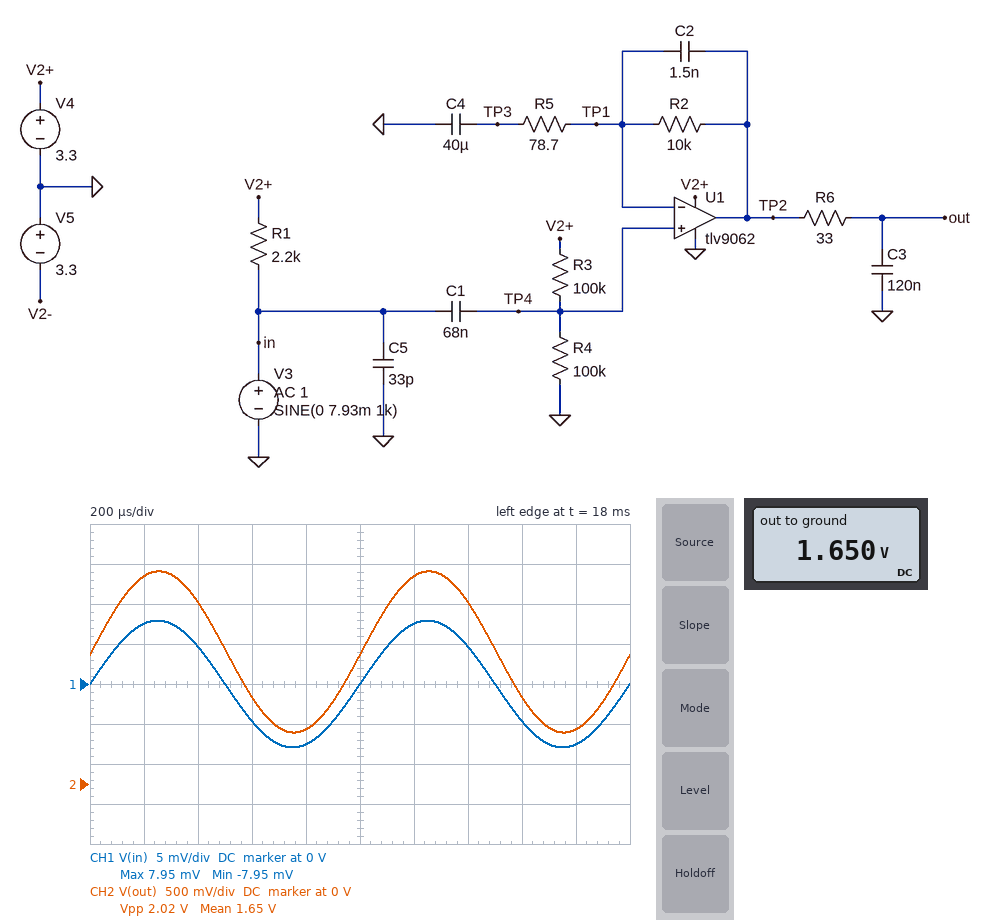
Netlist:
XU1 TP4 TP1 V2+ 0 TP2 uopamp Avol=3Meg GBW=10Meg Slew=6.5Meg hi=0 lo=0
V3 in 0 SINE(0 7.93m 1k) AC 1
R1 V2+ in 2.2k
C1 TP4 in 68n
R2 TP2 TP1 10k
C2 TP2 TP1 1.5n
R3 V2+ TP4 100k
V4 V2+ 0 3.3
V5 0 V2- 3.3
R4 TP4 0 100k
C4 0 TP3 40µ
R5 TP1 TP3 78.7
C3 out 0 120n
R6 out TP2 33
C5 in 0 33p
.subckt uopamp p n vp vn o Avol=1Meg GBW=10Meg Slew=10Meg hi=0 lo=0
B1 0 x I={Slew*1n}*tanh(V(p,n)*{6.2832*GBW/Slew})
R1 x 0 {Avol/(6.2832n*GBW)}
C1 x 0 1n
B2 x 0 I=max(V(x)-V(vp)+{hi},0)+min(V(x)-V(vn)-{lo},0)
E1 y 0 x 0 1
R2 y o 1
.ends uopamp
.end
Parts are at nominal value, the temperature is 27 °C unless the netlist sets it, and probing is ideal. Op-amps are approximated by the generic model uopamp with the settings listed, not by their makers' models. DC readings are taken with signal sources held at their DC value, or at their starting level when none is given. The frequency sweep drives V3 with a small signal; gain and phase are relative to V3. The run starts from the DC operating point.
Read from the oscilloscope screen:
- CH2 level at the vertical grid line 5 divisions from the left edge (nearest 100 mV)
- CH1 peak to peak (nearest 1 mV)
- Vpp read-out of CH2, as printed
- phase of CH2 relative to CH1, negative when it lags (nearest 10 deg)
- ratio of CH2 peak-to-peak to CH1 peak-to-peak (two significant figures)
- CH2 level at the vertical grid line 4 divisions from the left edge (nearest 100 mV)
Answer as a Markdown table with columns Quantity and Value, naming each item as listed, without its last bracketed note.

| Quantity | Value |
|---|---|
| CH2 level at the vertical grid line 5 divisions from the left edge | 1.6 V |
| CH1 peak to peak | 16 mV |
| Vpp read-out of CH2, as printed | 2.02 V |
| phase of CH2 relative to CH1, negative when it lags | 0 deg |
| ratio of CH2 peak-to-peak to CH1 peak-to-peak | 130 |
| CH2 level at the vertical grid line 4 divisions from the left edge | 700 mV |
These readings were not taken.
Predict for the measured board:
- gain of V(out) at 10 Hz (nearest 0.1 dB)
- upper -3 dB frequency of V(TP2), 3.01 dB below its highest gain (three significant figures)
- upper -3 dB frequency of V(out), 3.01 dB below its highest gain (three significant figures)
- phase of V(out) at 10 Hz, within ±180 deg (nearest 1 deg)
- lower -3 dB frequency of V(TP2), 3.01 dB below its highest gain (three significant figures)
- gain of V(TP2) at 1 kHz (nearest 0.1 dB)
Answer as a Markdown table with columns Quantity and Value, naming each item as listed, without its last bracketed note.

| Quantity | Value |
|---|---|
| gain of V(out) at 10 Hz | 14.3 dB |
| upper -3 dB frequency of V(TP2), 3.01 dB below its highest gain | 9.49 kHz |
| upper -3 dB frequency of V(out), 3.01 dB below its highest gain | 9.03 kHz |
| phase of V(out) at 10 Hz, within ±180 deg | 154 deg |
| lower -3 dB frequency of V(TP2), 3.01 dB below its highest gain | 74.8 Hz |
| gain of V(TP2) at 1 kHz | 42.1 dB |
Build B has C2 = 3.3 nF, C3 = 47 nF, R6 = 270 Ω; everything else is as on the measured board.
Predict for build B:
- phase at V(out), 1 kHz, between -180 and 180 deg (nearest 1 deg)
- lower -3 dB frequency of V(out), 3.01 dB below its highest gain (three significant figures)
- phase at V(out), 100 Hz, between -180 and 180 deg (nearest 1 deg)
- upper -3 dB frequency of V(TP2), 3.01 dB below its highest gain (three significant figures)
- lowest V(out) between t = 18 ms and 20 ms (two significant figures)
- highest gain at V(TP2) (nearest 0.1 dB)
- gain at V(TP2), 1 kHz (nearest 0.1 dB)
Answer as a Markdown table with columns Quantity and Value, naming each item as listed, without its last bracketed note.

| Quantity | Value |
|---|---|
| phase at V(out), 1 kHz, between -180 and 180 deg | -11 deg |
| lower -3 dB frequency of V(out), 3.01 dB below its highest gain | 73.7 Hz |
| phase at V(out), 100 Hz, between -180 and 180 deg | 50 deg |
| upper -3 dB frequency of V(TP2), 3.01 dB below its highest gain | 4.68 kHz |
| lowest V(out) between t = 18 ms and 20 ms | 660 mV |
| highest gain at V(TP2) | 42.0 dB |
| gain at V(TP2), 1 kHz | 41.9 dB |
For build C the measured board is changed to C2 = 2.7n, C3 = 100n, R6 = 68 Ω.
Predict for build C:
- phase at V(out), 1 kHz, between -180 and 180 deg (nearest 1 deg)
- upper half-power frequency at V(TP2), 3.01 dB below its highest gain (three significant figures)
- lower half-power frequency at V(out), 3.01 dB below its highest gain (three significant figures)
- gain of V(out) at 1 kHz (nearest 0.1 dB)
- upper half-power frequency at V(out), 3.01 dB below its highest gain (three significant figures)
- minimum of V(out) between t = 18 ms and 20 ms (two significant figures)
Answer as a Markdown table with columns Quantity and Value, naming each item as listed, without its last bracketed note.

| Quantity | Value |
|---|---|
| phase at V(out), 1 kHz, between -180 and 180 deg | -7 deg |
| upper half-power frequency at V(TP2), 3.01 dB below its highest gain | 5.62 kHz |
| lower half-power frequency at V(out), 3.01 dB below its highest gain | 74.1 Hz |
| gain of V(out) at 1 kHz | 42.0 dB |
| upper half-power frequency at V(out), 3.01 dB below its highest gain | 5.34 kHz |
| minimum of V(out) between t = 18 ms and 20 ms | 650 mV |
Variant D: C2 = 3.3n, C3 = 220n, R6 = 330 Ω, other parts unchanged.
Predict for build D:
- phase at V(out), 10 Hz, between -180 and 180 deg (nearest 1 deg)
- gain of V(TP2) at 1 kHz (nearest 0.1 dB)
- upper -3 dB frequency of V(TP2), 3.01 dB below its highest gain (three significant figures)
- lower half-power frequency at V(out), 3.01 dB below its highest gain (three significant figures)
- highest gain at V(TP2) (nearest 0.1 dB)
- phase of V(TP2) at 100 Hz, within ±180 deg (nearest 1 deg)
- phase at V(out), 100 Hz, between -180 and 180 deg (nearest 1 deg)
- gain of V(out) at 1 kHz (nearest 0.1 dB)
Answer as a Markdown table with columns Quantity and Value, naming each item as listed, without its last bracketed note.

| Quantity | Value |
|---|---|
| phase at V(out), 10 Hz, between -180 and 180 deg | 154 deg |
| gain of V(TP2) at 1 kHz | 41.9 dB |
| upper -3 dB frequency of V(TP2), 3.01 dB below its highest gain | 4.68 kHz |
| lower half-power frequency at V(out), 3.01 dB below its highest gain | 71.6 Hz |
| highest gain at V(TP2) | 42.0 dB |
| phase of V(TP2) at 100 Hz, within ±180 deg | 50 deg |
| phase at V(out), 100 Hz, between -180 and 180 deg | 48 deg |
| gain of V(out) at 1 kHz | 41.1 dB |
